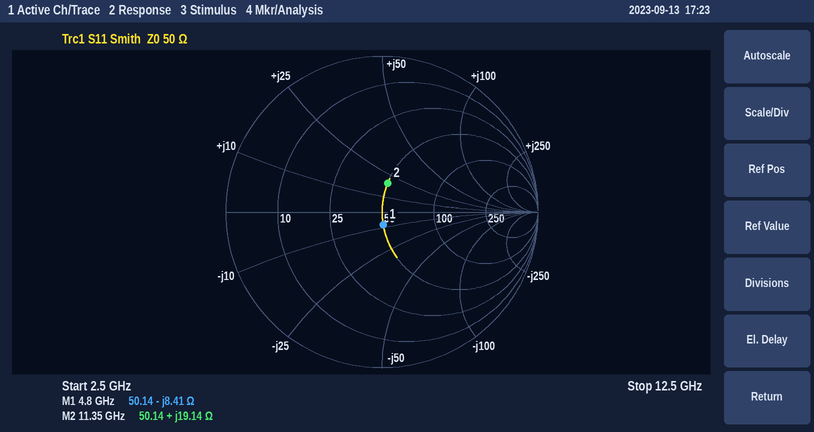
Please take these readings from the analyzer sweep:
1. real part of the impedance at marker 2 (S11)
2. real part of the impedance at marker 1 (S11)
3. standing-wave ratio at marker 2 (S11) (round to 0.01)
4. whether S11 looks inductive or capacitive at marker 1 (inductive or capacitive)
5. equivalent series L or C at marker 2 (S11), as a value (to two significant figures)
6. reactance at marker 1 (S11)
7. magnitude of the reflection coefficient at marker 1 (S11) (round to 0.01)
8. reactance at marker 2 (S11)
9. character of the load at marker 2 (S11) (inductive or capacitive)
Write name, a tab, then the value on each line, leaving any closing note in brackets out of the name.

real part of the impedance at marker 2	50.14 Ω
real part of the impedance at marker 1	50.14 Ω
standing-wave ratio at marker 2 (S11)	1.46
whether S11 looks inductive or capacitive at marker 1	capacitive
equivalent series L or C at marker 2 (S11), as a value	270 pH
reactance at marker 1	-8.41 Ω
magnitude of the reflection coefficient at marker 1 (S11)	0.08
reactance at marker 2	+19.14 Ω
character of the load at marker 2 (S11)	inductive
